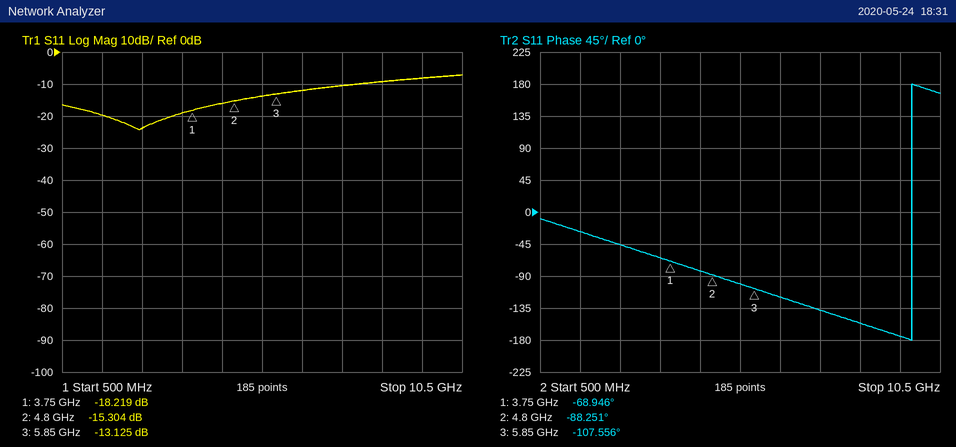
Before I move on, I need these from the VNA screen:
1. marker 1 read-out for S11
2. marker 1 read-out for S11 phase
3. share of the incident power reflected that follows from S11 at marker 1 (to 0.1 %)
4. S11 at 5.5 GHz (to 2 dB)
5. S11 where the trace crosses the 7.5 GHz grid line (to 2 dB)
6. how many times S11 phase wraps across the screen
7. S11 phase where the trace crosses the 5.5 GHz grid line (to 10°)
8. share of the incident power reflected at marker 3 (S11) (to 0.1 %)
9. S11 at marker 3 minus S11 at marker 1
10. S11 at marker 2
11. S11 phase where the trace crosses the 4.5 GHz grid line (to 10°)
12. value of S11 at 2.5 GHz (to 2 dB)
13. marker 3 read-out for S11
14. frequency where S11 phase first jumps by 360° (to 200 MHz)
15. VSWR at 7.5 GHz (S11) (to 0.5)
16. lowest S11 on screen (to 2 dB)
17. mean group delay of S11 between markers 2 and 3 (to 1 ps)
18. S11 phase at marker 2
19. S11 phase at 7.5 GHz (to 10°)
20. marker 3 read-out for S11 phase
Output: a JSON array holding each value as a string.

["-18.219 dB", "-68.946°", "1.5 %", "-14 dB", "-10 dB", "1", "-100°", "4.9 %", "5.094 dB", "-15.304 dB", "-80°", "-24 dB", "-13.125 dB", "9.8 GHz", "2.0", "-24 dB", "51 ps", "-88.251°", "-140°", "-107.556°"]
